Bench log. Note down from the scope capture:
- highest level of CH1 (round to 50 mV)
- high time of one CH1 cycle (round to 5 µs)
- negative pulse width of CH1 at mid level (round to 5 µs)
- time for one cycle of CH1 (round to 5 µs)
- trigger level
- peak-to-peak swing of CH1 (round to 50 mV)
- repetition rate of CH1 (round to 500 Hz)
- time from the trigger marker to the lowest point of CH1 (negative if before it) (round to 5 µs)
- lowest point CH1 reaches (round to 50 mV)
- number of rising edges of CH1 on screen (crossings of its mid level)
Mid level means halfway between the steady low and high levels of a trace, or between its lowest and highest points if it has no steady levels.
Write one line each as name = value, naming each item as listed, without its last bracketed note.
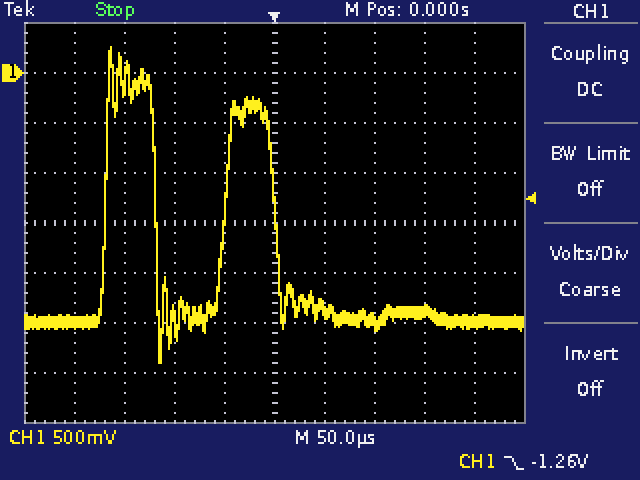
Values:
highest level of CH1 = 250 mV
high time of one CH1 cycle = 50 µs
negative pulse width of CH1 at mid level = 70 µs
time for one cycle of CH1 = 120 µs
trigger level = -1.26 V
peak-to-peak swing of CH1 = 3.15 V
repetition rate of CH1 = 8.5 kHz
time from the trigger marker to the lowest point of CH1 (negative if before it) = -115 µs
lowest point CH1 reaches = -2.90 V
number of rising edges of CH1 on screen = 2
